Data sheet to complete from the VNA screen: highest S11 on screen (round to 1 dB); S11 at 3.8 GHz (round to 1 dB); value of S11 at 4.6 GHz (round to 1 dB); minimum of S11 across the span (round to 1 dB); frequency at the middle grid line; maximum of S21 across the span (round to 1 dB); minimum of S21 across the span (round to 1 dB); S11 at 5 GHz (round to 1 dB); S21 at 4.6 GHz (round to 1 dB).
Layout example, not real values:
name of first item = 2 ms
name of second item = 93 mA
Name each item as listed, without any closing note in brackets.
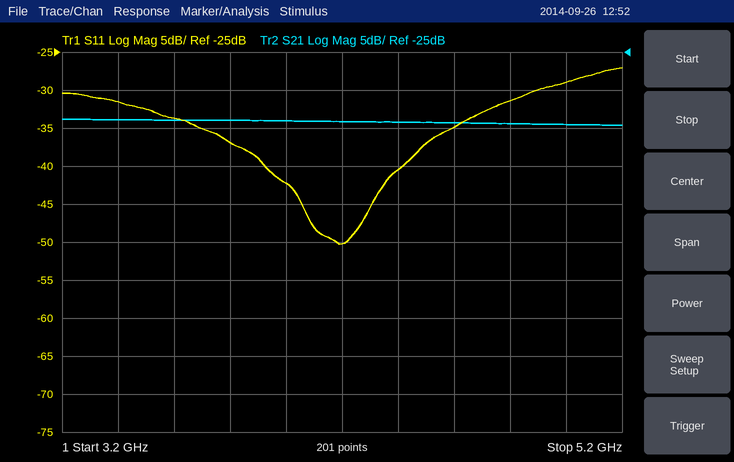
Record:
highest S11 on screen = -27 dB
S11 at 3.8 GHz = -37 dB
value of S11 at 4.6 GHz = -35 dB
minimum of S11 across the span = -50 dB
frequency at the middle grid line = 4.2 GHz
maximum of S21 across the span = -34 dB
minimum of S21 across the span = -35 dB
S11 at 5 GHz = -29 dB
S21 at 4.6 GHz = -34 dB
